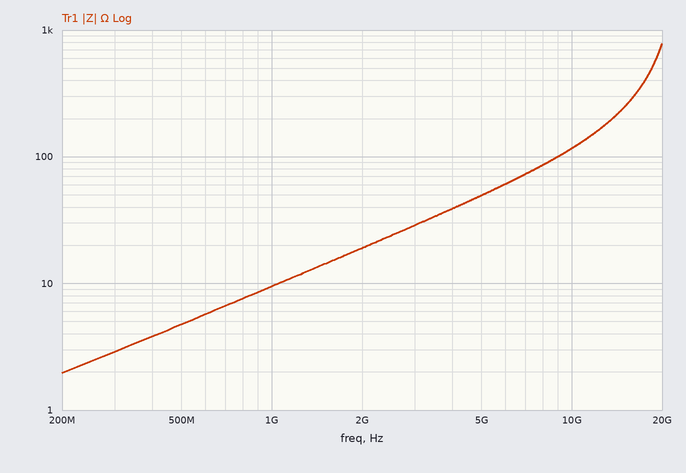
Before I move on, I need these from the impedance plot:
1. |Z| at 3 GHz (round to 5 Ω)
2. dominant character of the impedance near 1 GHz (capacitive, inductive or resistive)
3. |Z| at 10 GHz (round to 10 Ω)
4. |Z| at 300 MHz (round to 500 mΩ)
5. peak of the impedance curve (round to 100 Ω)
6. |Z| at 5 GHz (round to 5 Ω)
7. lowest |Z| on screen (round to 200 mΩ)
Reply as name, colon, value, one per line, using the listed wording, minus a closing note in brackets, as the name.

|Z| at 3 GHz: 30 Ω
dominant character of the impedance near 1 GHz: inductive
|Z| at 10 GHz: 120 Ω
|Z| at 300 MHz: 3.0 Ω
peak of the impedance curve: 800 Ω
|Z| at 5 GHz: 50 Ω
lowest |Z| on screen: 2.0 Ω
